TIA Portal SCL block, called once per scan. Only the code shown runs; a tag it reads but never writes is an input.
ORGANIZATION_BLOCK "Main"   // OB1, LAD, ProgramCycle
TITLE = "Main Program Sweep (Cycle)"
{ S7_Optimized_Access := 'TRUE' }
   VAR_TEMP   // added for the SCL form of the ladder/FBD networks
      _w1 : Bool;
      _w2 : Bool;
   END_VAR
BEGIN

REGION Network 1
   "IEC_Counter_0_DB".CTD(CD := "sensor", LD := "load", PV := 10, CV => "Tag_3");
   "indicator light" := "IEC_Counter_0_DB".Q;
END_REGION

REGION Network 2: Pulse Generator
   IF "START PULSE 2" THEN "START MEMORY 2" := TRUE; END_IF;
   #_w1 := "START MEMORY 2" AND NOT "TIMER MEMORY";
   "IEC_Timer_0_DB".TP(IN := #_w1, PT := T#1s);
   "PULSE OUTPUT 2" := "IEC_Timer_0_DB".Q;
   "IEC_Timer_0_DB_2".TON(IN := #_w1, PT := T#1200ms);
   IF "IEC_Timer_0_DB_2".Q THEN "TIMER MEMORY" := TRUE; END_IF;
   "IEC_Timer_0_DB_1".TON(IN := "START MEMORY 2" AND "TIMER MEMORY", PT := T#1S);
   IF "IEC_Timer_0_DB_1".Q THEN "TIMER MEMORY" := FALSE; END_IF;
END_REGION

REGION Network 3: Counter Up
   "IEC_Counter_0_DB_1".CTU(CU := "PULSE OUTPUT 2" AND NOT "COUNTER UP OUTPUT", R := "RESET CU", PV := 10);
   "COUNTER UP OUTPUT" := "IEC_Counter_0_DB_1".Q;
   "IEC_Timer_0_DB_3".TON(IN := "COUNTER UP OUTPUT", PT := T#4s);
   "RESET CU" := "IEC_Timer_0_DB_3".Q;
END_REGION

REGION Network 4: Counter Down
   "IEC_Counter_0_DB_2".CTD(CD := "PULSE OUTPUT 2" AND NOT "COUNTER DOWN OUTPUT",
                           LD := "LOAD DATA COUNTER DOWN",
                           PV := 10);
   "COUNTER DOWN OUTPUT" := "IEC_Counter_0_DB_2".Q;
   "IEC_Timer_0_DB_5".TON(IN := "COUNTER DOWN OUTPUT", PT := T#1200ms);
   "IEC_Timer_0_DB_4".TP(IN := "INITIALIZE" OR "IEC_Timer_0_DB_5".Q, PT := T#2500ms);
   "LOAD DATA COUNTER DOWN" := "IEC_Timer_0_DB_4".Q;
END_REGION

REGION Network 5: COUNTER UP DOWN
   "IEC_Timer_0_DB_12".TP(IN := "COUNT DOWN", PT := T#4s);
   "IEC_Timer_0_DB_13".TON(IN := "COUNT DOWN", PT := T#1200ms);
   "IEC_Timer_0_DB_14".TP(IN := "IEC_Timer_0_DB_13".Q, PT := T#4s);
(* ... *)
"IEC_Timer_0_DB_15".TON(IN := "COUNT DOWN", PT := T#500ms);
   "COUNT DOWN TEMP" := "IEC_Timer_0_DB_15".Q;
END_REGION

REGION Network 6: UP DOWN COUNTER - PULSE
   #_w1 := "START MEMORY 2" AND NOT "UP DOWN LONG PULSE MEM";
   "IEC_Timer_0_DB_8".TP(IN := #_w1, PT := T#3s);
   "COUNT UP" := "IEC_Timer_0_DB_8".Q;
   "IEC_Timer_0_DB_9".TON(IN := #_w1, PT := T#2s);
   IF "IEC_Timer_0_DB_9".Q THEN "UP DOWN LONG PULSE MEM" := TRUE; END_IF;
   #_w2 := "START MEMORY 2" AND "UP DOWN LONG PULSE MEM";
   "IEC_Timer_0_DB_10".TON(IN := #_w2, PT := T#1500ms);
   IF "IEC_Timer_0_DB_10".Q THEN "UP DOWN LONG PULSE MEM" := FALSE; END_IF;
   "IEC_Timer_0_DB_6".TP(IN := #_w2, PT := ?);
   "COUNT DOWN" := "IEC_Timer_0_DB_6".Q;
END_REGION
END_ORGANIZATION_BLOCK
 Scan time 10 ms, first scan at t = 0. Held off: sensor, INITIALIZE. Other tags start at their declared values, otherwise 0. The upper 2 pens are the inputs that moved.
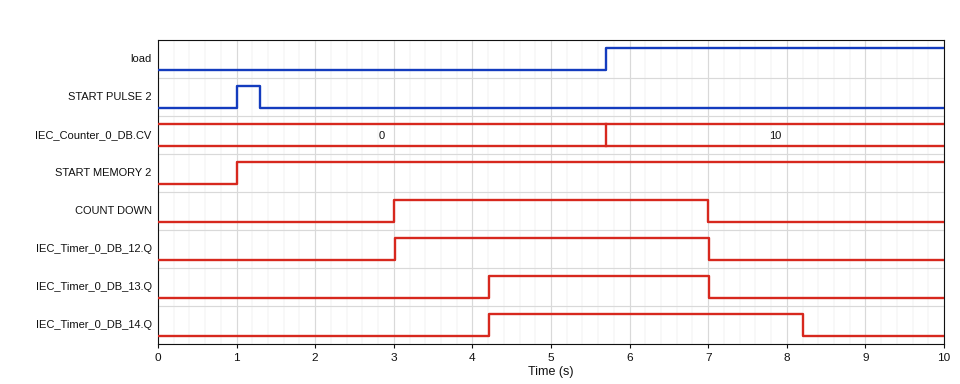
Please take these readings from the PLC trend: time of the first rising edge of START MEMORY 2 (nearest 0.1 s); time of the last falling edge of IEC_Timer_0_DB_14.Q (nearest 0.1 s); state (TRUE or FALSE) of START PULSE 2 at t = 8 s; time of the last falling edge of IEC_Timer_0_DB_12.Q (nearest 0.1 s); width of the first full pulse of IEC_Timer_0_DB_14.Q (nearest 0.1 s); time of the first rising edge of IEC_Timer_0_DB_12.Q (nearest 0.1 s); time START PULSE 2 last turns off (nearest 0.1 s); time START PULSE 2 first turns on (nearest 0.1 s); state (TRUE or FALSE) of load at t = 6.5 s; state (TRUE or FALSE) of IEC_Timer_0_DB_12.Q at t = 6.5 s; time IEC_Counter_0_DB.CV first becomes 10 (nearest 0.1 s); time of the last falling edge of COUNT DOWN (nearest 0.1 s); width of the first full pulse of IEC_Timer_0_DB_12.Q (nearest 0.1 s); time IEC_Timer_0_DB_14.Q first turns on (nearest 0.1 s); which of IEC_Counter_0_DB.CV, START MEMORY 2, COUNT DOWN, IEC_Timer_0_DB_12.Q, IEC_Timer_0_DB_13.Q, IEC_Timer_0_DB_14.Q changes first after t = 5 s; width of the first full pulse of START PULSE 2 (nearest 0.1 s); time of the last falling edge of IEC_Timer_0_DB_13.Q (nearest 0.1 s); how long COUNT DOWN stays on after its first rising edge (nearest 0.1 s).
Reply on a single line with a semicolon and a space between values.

1.0 s; 8.2 s; FALSE; 7.0 s; 4.0 s; 3.0 s; 1.3 s; 1.0 s; TRUE; TRUE; 5.7 s; 7.0 s; 4.0 s; 4.2 s; IEC_Counter_0_DB.CV; 0.3 s; 7.0 s; 4.0 s
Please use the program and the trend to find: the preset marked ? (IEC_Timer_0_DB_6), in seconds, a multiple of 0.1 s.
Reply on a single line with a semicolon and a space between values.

4.0 s
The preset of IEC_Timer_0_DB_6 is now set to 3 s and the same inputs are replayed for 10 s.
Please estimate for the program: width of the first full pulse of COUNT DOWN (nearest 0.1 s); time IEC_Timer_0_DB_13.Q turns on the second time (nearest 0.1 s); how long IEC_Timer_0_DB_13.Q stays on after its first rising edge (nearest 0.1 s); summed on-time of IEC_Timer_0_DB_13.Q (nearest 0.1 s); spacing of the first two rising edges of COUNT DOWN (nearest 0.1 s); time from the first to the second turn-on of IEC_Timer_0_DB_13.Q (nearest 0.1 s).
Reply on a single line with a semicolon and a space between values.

3.0 s; 7.7 s; 1.8 s; 3.6 s; 3.5 s; 3.5 s
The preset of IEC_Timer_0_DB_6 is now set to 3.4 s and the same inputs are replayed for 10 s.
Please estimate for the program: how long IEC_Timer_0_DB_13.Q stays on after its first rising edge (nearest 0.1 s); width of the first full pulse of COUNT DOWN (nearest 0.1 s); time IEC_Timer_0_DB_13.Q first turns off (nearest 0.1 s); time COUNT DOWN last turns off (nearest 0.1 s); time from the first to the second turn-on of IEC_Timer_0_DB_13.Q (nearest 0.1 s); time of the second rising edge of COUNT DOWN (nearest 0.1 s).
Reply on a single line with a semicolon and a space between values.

2.2 s; 3.4 s; 6.4 s; 9.9 s; 3.5 s; 6.5 s
